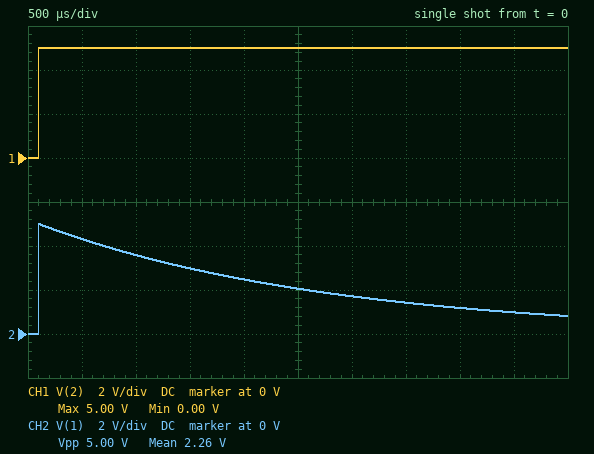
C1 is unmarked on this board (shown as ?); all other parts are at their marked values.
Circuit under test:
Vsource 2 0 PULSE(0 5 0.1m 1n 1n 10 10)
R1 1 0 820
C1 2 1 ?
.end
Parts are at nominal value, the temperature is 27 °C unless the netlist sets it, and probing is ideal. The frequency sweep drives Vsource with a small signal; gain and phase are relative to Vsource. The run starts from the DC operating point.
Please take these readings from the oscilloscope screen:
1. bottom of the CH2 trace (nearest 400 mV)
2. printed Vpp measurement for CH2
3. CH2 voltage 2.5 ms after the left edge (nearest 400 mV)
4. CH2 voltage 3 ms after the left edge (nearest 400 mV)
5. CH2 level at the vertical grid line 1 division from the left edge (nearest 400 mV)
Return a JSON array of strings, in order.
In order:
["0 V", "5.00 V", "2.0 V", "1.6 V", "4.4 V"]
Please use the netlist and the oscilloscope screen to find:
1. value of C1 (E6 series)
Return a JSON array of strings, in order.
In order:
["3.3 µF"]
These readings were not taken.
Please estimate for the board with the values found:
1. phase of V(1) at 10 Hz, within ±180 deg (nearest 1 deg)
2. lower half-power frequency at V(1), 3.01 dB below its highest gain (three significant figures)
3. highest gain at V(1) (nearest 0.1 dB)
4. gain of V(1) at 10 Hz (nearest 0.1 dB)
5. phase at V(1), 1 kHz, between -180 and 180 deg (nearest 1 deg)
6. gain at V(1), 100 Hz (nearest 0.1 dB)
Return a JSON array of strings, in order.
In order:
["80 deg", "58.8 Hz", "0 dB", "-15.5 dB", "3 deg", "-1.3 dB"]
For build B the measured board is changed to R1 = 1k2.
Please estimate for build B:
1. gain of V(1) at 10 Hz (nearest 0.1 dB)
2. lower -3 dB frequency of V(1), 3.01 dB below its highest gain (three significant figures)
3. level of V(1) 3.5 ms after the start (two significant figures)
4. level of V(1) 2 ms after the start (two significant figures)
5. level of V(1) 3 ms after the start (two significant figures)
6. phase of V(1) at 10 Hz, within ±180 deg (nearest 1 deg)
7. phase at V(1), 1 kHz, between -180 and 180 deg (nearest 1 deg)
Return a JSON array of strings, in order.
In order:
["-12.3 dB", "40.2 Hz", "2.1 V", "3.1 V", "2.4 V", "76 deg", "2 deg"]
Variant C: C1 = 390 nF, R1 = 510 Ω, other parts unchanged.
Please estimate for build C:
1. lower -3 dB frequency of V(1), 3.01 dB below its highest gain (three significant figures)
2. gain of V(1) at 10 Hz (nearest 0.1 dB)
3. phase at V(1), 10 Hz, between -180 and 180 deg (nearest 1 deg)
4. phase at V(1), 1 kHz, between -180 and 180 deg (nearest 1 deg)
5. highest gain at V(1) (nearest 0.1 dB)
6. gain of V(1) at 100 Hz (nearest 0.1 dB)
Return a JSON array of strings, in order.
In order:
["800 Hz", "-38.1 dB", "89 deg", "39 deg", "0 dB", "-18.1 dB"]
